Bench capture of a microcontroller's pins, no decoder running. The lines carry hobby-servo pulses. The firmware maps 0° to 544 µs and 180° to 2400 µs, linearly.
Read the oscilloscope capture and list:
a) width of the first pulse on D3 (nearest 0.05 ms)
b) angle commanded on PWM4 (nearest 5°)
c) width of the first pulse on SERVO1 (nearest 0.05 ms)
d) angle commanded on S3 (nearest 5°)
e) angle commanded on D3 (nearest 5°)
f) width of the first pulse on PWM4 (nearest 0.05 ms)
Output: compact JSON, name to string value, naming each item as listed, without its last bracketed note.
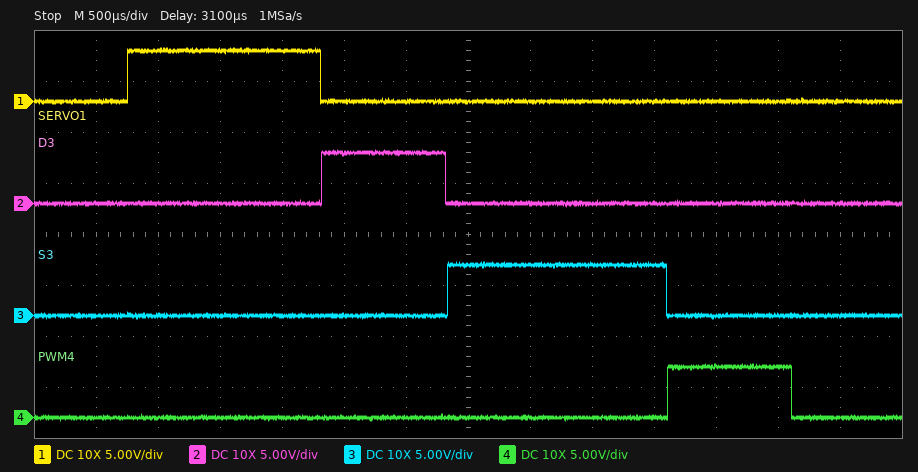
{"width of the first pulse on D3": "1.00 ms", "angle commanded on PWM4": "45°", "width of the first pulse on SERVO1": "1.55 ms", "angle commanded on S3": "120°", "angle commanded on D3": "45°", "width of the first pulse on PWM4": "1.00 ms"}
